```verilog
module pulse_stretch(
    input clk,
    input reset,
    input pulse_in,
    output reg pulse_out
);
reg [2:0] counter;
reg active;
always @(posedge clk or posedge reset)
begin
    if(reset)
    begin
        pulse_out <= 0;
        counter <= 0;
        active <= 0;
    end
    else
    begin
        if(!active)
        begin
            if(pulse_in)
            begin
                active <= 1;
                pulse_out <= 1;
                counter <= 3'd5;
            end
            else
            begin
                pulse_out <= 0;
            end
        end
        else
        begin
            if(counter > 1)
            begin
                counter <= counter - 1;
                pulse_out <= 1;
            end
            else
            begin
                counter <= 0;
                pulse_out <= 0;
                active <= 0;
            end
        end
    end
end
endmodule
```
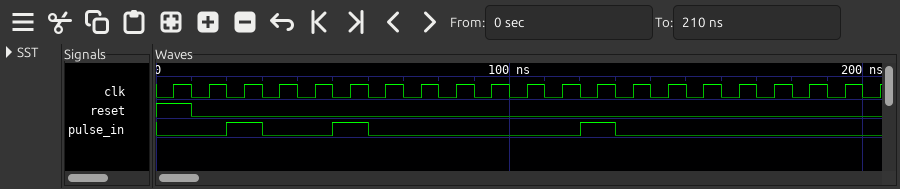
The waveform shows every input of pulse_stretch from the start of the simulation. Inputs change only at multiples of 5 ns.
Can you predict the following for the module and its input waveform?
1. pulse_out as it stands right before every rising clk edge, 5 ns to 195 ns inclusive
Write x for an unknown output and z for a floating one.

0 0 0 1 1 1 1 1 0 0 0 0 0 1 1 1 1 1 0 0
